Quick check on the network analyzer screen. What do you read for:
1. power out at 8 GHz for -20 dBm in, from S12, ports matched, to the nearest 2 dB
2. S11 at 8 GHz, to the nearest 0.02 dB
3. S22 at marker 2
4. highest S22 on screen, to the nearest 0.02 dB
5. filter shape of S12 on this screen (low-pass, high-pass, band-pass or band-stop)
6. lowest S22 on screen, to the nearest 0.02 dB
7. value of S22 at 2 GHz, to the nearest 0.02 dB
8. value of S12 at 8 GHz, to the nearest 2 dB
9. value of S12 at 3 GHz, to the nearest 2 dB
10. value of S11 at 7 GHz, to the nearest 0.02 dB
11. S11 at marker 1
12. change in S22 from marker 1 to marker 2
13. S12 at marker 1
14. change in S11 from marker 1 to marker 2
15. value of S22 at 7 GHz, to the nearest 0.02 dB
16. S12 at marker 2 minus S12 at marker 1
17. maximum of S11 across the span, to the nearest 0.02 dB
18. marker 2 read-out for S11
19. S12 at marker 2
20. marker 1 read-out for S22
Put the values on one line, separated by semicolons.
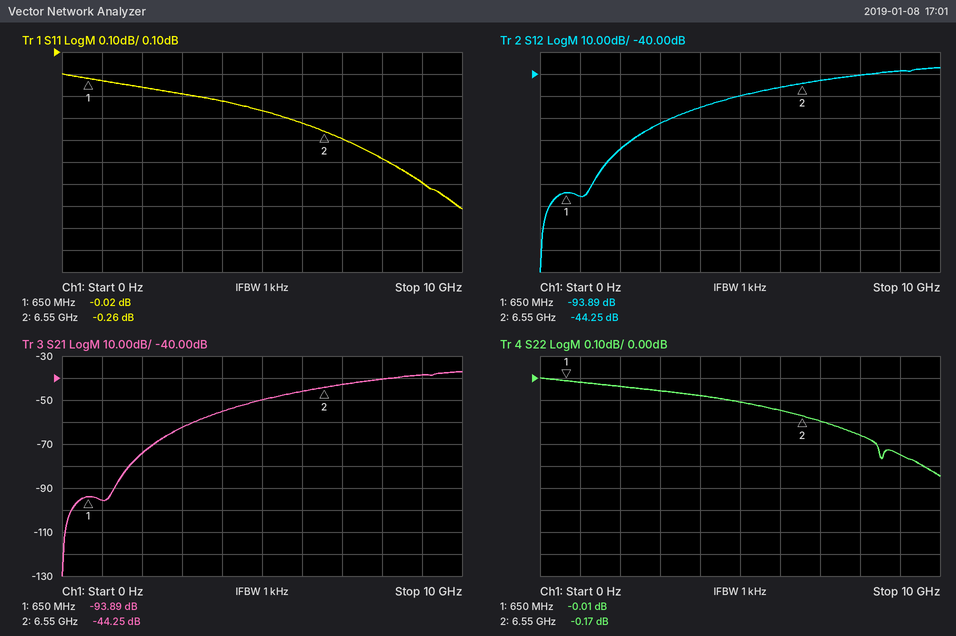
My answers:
-60 dBm; -0.38 dB; -0.17 dB; 0.00 dB; high-pass; -0.44 dB; -0.04 dB; -40 dB; -62 dB; -0.30 dB; -0.02 dB; -0.16 dB; -93.89 dB; -0.24 dB; -0.20 dB; 49.64 dB; 0.00 dB; -0.26 dB; -44.25 dB; -0.01 dB
